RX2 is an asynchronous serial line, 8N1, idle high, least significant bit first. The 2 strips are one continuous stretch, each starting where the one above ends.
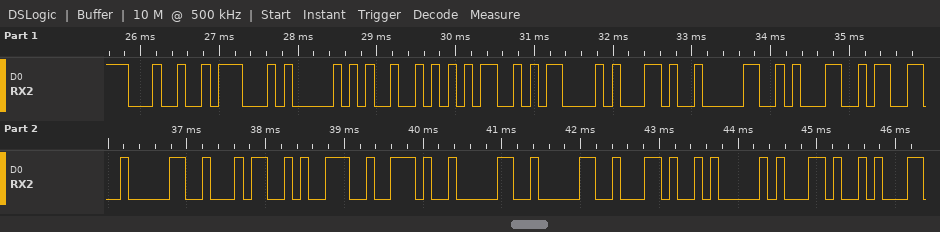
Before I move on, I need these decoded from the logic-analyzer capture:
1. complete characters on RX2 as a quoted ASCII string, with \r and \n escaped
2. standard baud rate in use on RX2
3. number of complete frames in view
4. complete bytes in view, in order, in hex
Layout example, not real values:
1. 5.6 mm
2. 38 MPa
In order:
1. "$GPRMC,013049.00,A,"
2. 9600 baud
3. 19
4. 0x24 0x47 0x50 0x52 0x4D 0x43 0x2C 0x30 0x31 0x33 0x30 0x34 0x39 0x2E 0x30 0x30 0x2C 0x41 0x2C
